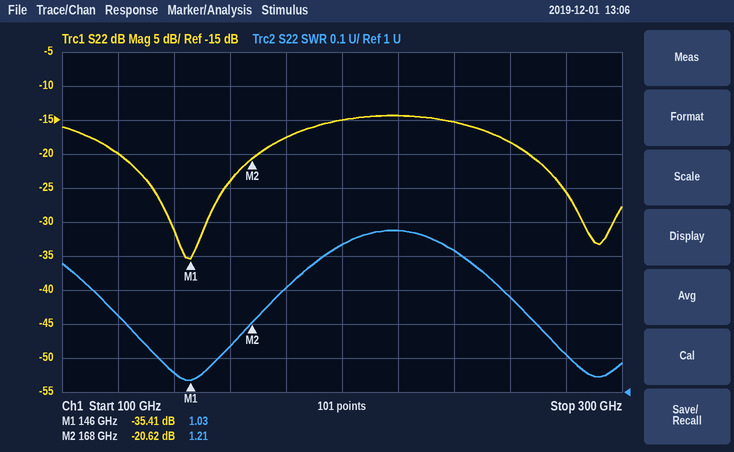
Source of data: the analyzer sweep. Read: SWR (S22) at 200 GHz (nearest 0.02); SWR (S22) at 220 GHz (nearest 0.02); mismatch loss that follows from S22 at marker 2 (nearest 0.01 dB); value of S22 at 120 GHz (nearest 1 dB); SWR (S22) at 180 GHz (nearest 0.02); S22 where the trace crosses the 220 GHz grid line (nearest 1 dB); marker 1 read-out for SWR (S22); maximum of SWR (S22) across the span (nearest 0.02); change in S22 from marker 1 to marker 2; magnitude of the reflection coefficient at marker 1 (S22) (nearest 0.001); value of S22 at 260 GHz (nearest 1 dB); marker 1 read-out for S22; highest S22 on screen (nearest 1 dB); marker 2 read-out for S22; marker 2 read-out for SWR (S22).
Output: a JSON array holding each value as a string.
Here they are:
["1.44", "1.48", "0.04 dB", "-20 dB", "1.30", "-14 dB", "1.03", "1.48", "14.79 dB", "0.017", "-18 dB", "-35.41 dB", "-14 dB", "-20.62 dB", "1.21"]
